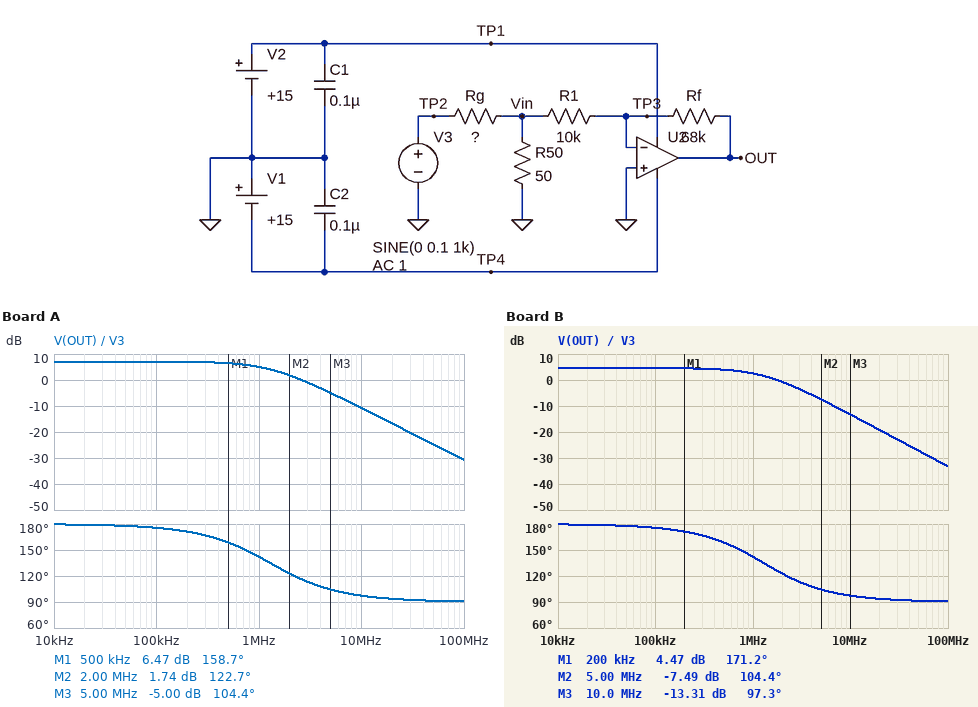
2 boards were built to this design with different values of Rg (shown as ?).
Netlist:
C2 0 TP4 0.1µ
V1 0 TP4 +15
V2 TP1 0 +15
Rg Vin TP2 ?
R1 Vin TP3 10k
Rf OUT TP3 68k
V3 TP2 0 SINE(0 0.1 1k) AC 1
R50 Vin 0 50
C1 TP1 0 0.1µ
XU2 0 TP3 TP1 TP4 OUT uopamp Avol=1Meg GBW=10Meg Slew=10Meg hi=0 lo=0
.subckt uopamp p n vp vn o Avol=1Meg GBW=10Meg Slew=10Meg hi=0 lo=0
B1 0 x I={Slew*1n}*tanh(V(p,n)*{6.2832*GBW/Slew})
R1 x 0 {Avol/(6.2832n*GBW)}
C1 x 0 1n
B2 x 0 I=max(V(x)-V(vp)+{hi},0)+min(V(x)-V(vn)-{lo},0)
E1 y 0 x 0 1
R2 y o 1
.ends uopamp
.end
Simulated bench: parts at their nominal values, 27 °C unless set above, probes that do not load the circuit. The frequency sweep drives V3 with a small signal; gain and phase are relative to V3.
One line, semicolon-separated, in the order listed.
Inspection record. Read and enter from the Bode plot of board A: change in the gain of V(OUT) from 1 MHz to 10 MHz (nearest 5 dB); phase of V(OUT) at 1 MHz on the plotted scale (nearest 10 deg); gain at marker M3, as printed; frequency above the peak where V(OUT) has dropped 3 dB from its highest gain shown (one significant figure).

-15 dB; 140 deg; -5.00 dB; 1 MHz
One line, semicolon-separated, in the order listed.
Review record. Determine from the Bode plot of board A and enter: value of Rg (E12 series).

100 Ω
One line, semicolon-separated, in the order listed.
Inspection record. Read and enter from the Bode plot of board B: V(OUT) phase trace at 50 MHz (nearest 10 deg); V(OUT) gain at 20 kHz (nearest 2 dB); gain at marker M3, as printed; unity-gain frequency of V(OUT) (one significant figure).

90 deg; 4 dB; -13.31 dB; 2 MHz
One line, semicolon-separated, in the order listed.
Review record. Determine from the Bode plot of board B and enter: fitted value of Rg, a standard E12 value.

150 Ω
